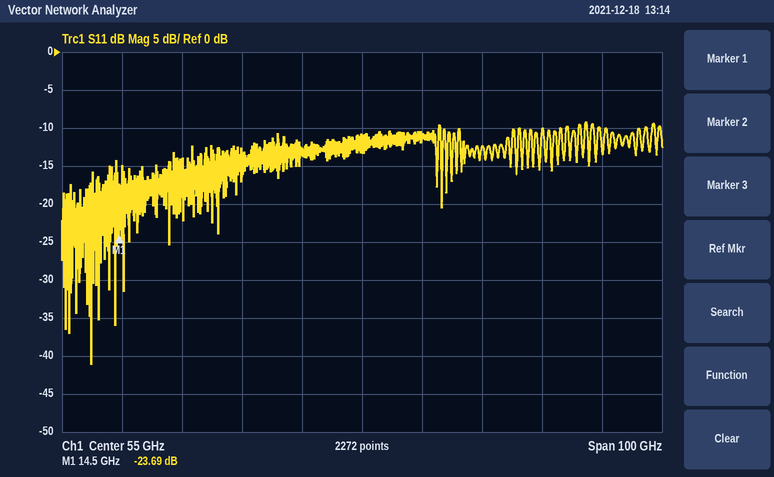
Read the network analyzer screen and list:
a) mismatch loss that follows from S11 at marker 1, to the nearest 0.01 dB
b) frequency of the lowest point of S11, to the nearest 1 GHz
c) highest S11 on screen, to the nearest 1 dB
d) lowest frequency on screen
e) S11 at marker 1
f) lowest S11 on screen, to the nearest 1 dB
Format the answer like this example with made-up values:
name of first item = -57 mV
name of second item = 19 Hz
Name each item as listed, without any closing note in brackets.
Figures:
mismatch loss that follows from S11 at marker 1, to the nearest 0.01 dB = 0.02 dB
frequency of the lowest point of S11, to the nearest 1 GHz = 10 GHz
highest S11 on screen, to the nearest 1 dB = -9 dB
lowest frequency on screen = 5 GHz
S11 at marker 1 = -23.69 dB
lowest S11 on screen, to the nearest 1 dB = -41 dB
